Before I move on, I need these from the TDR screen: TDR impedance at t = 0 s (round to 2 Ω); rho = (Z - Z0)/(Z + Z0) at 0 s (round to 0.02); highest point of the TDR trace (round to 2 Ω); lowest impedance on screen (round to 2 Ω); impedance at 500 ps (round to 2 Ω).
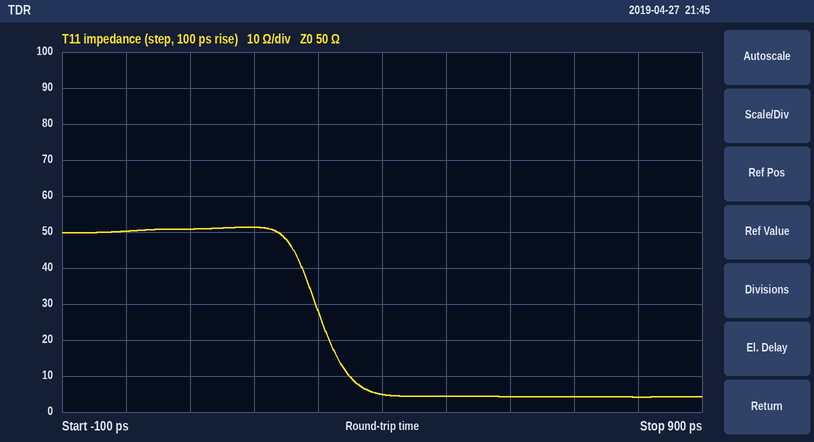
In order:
50 Ω
0.00
52 Ω
4 Ω
4 Ω
